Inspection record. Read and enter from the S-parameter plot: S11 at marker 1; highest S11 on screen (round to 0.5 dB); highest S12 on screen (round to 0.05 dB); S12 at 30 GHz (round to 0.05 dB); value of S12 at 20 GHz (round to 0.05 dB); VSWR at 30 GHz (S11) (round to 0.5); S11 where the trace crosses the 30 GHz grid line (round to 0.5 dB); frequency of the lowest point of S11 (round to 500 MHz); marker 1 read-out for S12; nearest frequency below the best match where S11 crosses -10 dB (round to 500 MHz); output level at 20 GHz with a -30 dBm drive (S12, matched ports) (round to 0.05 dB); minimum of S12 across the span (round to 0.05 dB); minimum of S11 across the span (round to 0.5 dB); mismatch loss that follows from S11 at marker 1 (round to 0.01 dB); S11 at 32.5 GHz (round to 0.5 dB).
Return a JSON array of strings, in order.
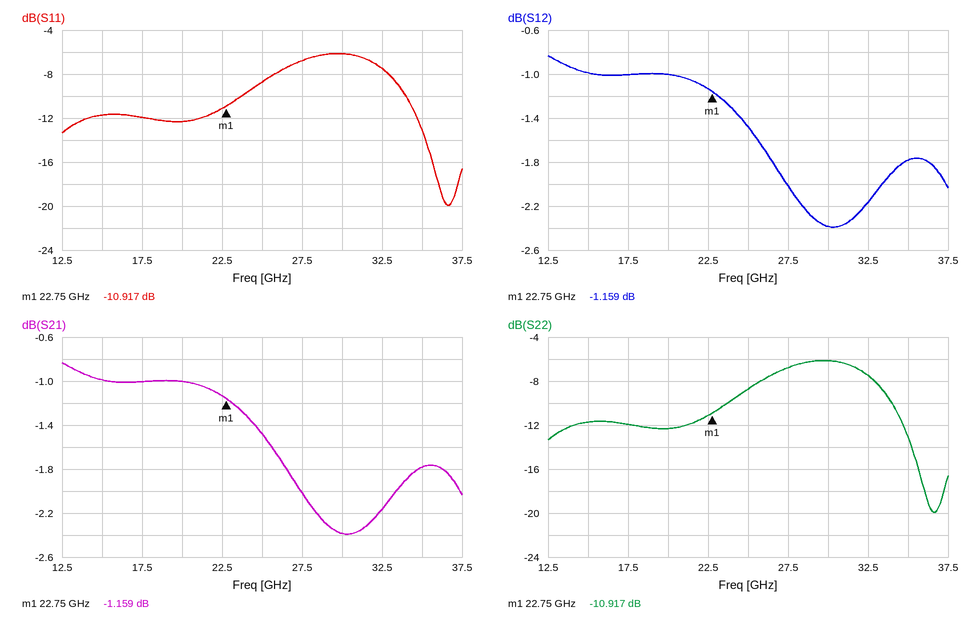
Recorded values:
["-10.917 dB", "-6.0 dB", "-0.85 dB", "-2.40 dB", "-1.00 dB", "3.0", "-6.0 dB", "36.5 GHz", "-1.159 dB", "34.0 GHz", "-31.00 dBm", "-2.40 dB", "-20.0 dB", "0.37 dB", "-7.5 dB"]
